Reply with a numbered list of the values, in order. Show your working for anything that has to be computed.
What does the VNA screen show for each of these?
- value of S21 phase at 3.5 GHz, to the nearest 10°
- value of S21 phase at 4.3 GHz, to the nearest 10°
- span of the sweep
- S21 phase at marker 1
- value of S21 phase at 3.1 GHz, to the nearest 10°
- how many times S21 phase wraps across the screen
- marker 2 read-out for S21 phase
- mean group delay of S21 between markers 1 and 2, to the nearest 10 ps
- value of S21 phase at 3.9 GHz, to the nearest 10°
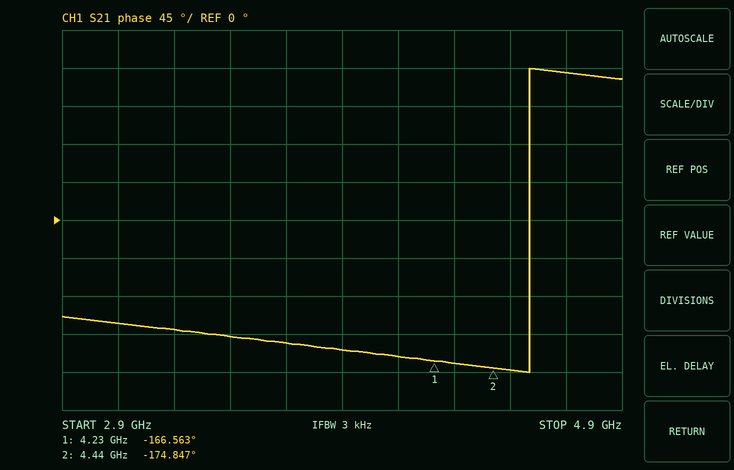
1. -140°
2. -170°
3. 2 GHz
4. -166.563°
5. -120°
6. 1
7. -174.847°
8. −(-174.847° − (-166.563°))/(360° × 210 MHz) ≈ 110 ps
9. -150°
